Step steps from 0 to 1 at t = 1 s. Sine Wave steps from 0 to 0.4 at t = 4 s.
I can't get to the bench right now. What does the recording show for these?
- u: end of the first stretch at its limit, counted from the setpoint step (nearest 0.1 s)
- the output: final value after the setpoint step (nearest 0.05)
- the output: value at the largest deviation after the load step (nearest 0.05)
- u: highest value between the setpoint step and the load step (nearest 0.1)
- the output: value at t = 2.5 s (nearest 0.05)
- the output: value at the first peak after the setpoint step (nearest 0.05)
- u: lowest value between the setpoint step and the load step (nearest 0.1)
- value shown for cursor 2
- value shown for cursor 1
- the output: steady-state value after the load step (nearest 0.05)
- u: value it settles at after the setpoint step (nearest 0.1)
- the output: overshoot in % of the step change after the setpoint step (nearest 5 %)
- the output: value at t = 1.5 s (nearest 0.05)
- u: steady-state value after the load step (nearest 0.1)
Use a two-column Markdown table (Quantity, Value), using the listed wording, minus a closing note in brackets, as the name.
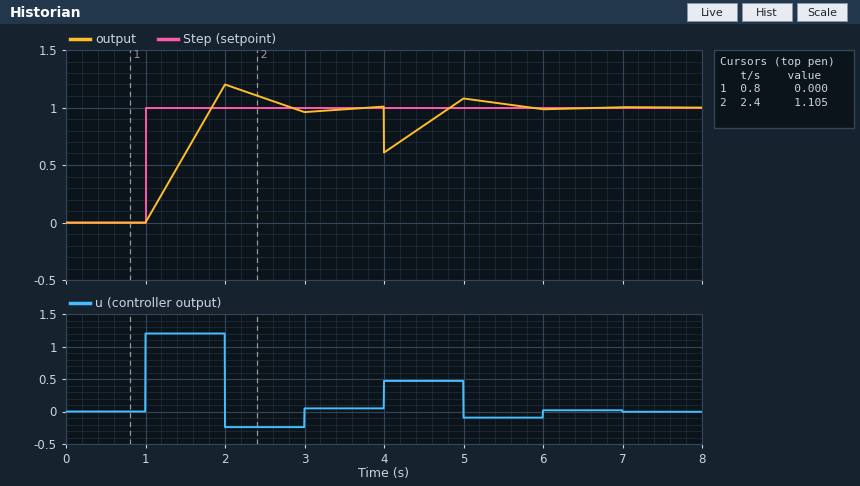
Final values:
| Quantity | Value |
|---|---|
| u: end of the first stretch at its limit, counted from the setpoint step | 1.0 s |
| the output: final value after the setpoint step | 1.00 |
| the output: value at the largest deviation after the load step | 0.60 |
| u: highest value between the setpoint step and the load step | 1.2 |
| the output: value at t = 2.5 s | 1.10 |
| the output: value at the first peak after the setpoint step | 1.20 |
| u: lowest value between the setpoint step and the load step | -0.2 |
| value shown for cursor 2 | 1.105 |
| value shown for cursor 1 | 0.000 |
| the output: steady-state value after the load step | 1.00 |
| u: value it settles at after the setpoint step | 0.0 |
| the output: overshoot in % of the step change after the setpoint step | 20 % |
| the output: value at t = 1.5 s | 0.60 |
| u: steady-state value after the load step | 0.0 |
